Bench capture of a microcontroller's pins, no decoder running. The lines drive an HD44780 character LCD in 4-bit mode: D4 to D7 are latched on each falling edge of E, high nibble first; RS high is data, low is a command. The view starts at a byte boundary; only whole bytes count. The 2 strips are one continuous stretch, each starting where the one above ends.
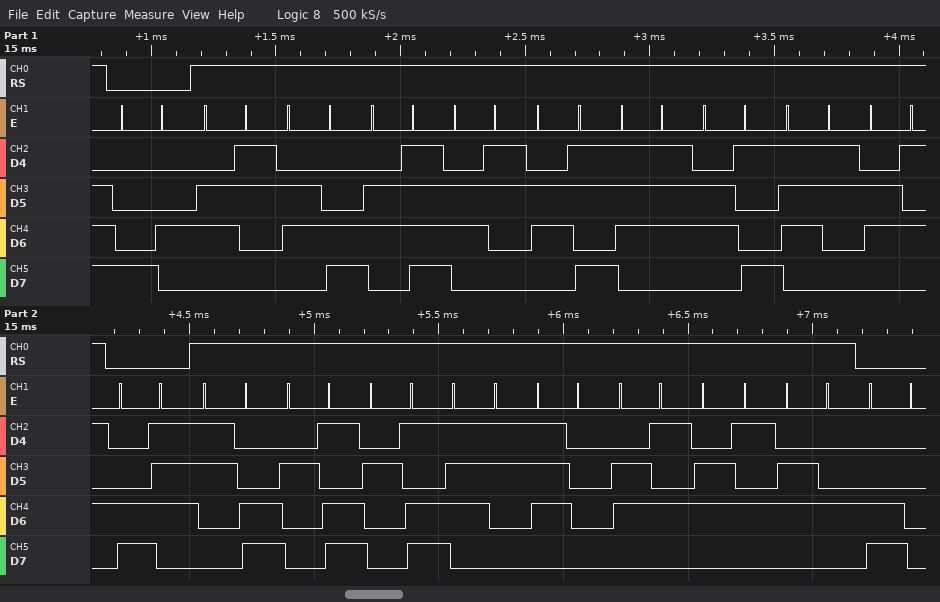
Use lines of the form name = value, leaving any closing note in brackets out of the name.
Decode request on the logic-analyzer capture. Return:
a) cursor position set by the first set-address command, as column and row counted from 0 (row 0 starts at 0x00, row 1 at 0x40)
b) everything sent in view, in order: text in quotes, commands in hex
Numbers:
cursor position set by the first set-address command, as column and row counted from 0 = column 4, row 0
everything sent in view, in order: text in quotes, commands in hex = 0x84 "clockwise" 0xC7 "<--speed" 0xC0
